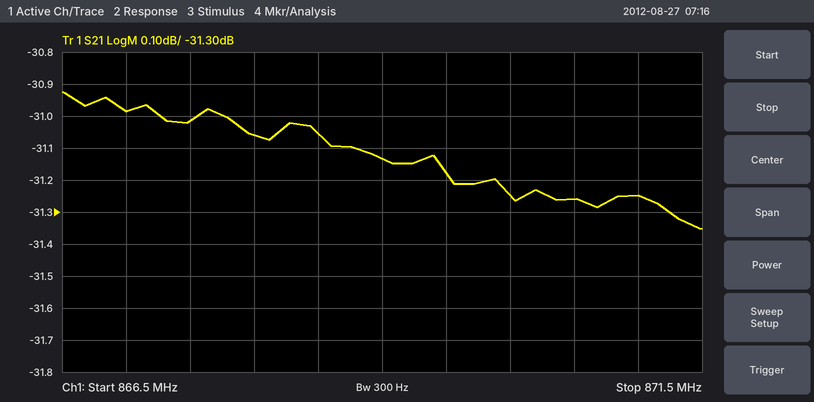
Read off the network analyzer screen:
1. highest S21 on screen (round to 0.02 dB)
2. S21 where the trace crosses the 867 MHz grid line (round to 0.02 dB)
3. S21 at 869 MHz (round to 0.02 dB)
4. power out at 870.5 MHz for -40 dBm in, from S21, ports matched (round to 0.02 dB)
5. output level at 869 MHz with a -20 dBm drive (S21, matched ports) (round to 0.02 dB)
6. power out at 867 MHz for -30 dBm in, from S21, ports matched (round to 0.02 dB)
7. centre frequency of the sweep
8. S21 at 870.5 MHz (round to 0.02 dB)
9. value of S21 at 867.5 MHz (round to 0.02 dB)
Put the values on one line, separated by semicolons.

-30.92 dB; -30.98 dB; -31.14 dB; -71.26 dBm; -51.14 dBm; -60.98 dBm; 869 MHz; -31.26 dB; -31.02 dB
